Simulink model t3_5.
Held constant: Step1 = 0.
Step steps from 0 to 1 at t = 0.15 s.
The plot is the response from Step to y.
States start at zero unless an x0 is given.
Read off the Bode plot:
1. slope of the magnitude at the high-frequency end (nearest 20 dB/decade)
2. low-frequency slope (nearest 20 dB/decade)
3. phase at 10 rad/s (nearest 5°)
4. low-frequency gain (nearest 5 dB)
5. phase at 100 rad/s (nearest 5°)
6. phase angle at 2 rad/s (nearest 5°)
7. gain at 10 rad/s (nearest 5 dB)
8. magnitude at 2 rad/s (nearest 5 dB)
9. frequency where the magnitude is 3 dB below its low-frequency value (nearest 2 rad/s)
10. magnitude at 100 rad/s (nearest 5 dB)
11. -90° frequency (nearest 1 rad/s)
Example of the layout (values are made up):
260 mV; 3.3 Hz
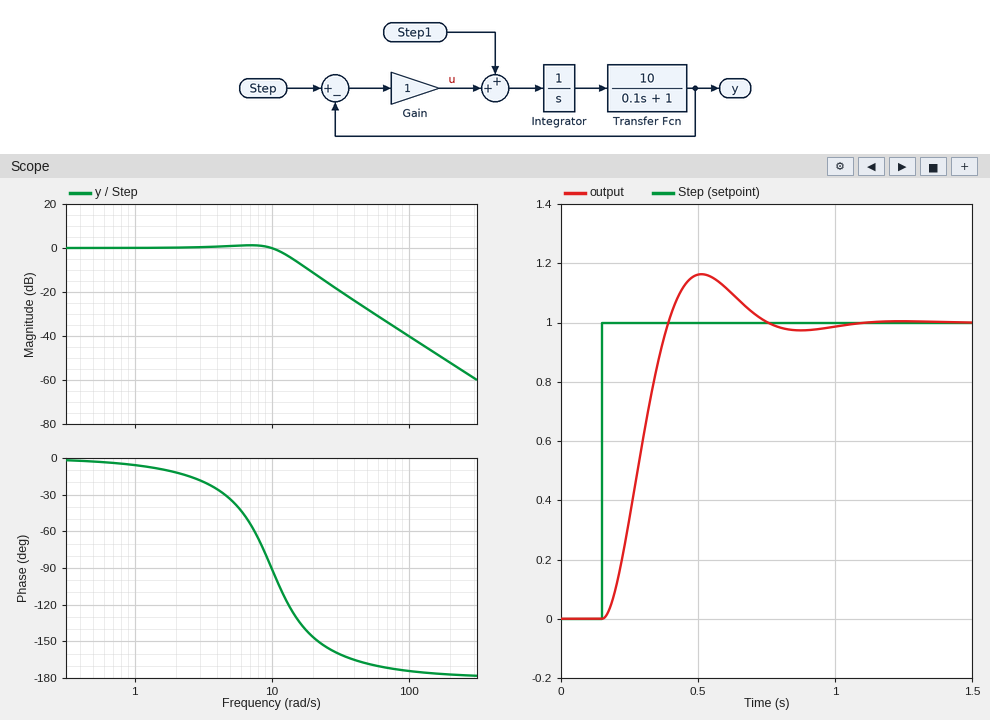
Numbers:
-40 dB/decade; 0 dB/decade; -90°; 0 dB; -175°; -10°; 0 dB; 0 dB; 12 rad/s; -40 dB; 10 rad/s
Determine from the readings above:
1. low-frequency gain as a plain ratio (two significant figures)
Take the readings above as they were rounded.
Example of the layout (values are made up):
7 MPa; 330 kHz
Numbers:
1.0
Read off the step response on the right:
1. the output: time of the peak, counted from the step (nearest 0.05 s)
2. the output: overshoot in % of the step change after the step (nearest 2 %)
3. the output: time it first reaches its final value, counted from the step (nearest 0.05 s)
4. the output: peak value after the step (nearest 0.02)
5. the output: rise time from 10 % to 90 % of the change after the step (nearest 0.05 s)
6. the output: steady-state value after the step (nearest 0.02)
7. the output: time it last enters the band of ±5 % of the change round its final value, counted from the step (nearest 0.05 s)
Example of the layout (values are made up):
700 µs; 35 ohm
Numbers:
0.35 s; 16 %; 0.25 s; 1.16; 0.15 s; 1.00; 0.55 s
